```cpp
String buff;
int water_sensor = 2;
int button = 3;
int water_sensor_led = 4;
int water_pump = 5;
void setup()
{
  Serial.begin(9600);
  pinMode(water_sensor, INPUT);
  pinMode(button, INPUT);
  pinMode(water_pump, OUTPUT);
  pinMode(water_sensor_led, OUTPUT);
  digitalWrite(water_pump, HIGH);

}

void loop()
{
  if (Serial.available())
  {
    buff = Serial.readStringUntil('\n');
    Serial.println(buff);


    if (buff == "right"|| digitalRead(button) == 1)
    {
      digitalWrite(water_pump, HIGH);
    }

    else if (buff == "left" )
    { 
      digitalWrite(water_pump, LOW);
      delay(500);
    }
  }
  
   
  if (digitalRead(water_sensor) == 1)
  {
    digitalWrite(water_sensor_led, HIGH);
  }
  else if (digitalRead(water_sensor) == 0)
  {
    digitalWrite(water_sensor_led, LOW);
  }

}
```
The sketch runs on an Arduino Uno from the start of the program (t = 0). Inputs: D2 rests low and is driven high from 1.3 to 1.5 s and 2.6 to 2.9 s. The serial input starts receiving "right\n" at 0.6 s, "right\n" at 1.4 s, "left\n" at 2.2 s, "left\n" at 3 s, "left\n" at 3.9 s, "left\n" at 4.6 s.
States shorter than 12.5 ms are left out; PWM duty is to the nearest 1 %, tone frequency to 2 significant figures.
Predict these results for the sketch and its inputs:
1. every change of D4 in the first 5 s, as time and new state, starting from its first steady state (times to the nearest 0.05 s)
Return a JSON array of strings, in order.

["0 s low; 1.3 s high; 1.5 s low; 2.7 s high; 2.9 s low"]
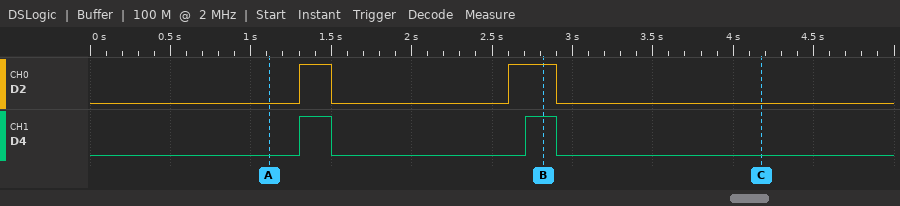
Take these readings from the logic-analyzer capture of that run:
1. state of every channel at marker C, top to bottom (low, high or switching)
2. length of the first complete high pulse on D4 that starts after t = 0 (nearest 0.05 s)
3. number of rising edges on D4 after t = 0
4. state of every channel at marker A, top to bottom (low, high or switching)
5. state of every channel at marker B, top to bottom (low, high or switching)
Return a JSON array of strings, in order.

["D2 low, D4 low", "0.20 s", "2", "D2 low, D4 low", "D2 high, D4 high"]
